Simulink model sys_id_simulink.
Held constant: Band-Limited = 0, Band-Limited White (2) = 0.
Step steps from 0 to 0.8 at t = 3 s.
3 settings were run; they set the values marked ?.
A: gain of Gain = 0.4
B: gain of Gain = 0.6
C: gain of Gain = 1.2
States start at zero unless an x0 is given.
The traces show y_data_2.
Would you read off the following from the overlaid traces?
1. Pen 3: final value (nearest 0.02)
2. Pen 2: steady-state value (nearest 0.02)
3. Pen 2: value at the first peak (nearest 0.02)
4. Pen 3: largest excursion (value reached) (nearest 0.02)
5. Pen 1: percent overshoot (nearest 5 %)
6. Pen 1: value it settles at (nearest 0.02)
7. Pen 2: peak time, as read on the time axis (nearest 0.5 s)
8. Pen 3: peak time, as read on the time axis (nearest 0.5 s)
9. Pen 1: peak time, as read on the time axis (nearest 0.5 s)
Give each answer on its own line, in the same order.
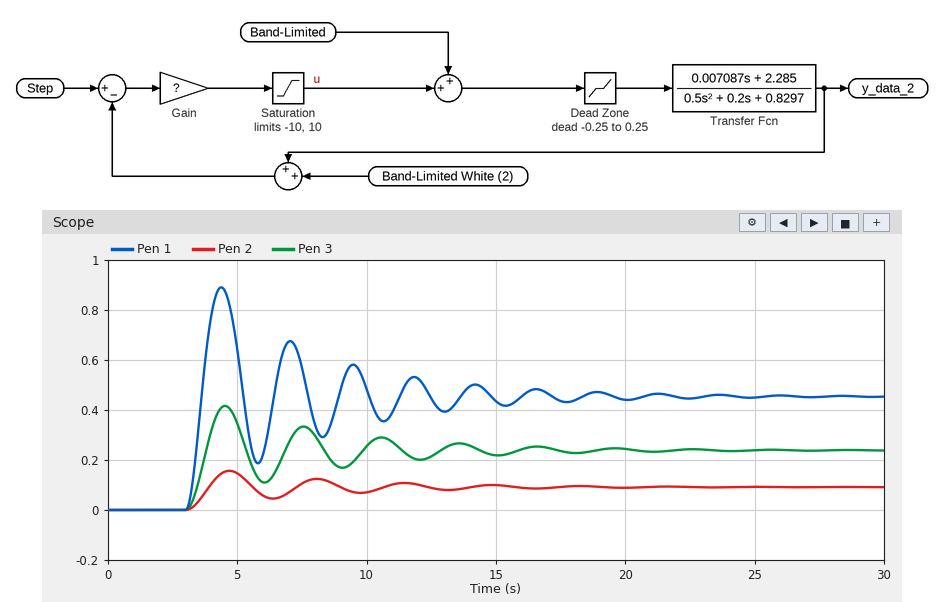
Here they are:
0.24
0.10
0.16
0.42
95 %
0.46
4.5 s
4.5 s
4.5 s
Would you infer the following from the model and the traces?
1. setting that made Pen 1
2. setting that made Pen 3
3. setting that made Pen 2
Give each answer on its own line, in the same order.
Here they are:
C
B
A
